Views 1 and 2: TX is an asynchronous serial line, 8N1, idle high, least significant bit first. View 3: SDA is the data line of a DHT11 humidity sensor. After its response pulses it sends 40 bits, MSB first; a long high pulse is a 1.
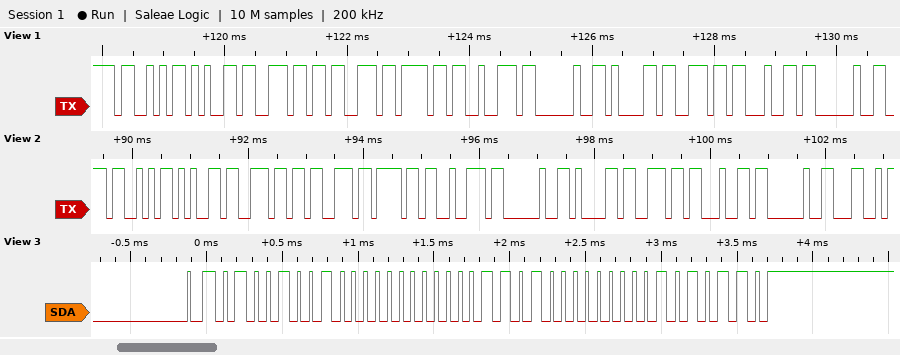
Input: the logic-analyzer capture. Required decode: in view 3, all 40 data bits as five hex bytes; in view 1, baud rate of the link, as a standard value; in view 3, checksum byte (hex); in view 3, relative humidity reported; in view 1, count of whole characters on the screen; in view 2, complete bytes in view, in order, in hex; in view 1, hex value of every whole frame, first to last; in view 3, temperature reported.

49 00 0D 00 56
9600 baud
0x56
73 %
11
53 65 6E 73 6F 72 20 61 6E 64 20 4C
53 65 6E 73 6F 72 20 61 6E 64 20
13.0 °C
